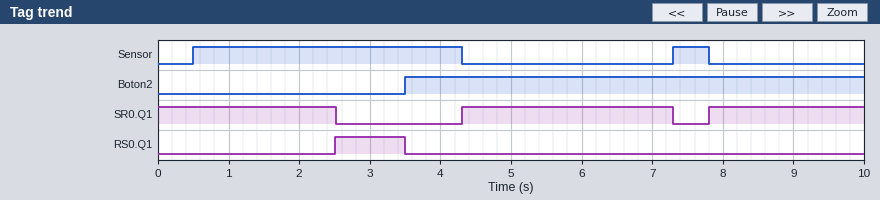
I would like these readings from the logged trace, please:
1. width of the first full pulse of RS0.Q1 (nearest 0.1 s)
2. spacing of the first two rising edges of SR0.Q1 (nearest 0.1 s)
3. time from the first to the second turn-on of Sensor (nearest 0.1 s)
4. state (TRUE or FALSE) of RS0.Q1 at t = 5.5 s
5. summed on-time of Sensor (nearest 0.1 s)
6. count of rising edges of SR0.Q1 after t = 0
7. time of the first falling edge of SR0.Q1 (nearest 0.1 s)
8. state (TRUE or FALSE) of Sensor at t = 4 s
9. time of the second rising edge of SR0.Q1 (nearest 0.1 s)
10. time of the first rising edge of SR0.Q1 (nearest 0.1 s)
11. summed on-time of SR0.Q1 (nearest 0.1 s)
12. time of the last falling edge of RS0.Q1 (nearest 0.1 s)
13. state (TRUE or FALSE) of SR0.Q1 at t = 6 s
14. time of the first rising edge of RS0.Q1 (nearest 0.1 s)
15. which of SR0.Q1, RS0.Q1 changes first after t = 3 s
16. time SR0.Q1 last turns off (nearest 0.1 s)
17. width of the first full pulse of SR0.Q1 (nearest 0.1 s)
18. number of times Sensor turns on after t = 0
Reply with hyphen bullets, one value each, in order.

- 1.0 s
- 3.5 s
- 6.8 s
- FALSE
- 4.3 s
- 2
- 2.5 s
- TRUE
- 7.8 s
- 4.3 s
- 7.7 s
- 3.5 s
- TRUE
- 2.5 s
- RS0.Q1
- 7.3 s
- 3.0 s
- 2
